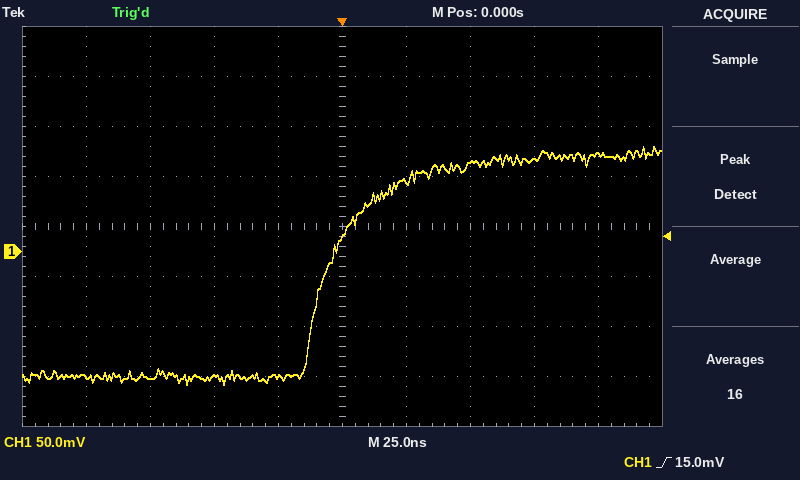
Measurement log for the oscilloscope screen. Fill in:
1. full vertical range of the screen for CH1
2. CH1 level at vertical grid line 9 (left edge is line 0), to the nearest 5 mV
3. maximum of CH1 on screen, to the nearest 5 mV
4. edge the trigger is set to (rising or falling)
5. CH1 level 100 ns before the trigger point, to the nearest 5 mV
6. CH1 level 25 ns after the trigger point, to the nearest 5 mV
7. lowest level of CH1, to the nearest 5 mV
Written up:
400 mV
95 mV
105 mV
rising
-125 mV
70 mV
-135 mV
